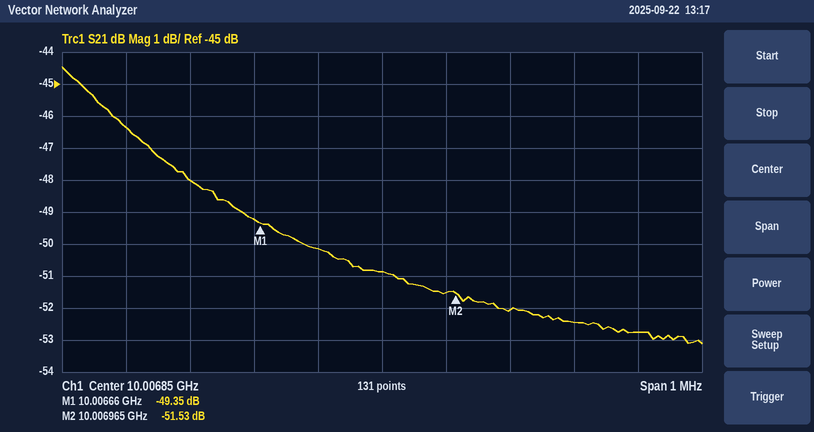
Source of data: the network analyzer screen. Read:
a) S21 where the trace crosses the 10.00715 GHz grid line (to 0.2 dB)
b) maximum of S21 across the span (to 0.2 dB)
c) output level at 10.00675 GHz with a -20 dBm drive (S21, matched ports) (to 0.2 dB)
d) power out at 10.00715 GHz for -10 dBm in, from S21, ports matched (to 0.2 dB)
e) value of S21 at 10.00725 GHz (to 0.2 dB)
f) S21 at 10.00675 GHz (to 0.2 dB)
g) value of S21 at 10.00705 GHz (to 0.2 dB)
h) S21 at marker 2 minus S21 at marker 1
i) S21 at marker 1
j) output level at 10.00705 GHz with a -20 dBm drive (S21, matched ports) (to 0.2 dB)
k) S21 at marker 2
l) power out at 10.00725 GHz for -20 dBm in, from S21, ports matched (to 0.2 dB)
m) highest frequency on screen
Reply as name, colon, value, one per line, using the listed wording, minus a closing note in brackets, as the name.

S21 where the trace crosses the 10.00715 GHz grid line: -52.4 dB
maximum of S21 across the span: -44.4 dB
output level at 10.00675 GHz with a -20 dBm drive (S21, matched ports): -70.2 dBm
power out at 10.00715 GHz for -10 dBm in, from S21, ports matched: -62.4 dBm
value of S21 at 10.00725 GHz: -52.8 dB
S21 at 10.00675 GHz: -50.2 dB
value of S21 at 10.00705 GHz: -52.0 dB
S21 at marker 2 minus S21 at marker 1: -2.18 dB
S21 at marker 1: -49.35 dB
output level at 10.00705 GHz with a -20 dBm drive (S21, matched ports): -72.0 dBm
S21 at marker 2: -51.53 dB
power out at 10.00725 GHz for -20 dBm in, from S21, ports matched: -72.8 dBm
highest frequency on screen: 10.00735 GHz
